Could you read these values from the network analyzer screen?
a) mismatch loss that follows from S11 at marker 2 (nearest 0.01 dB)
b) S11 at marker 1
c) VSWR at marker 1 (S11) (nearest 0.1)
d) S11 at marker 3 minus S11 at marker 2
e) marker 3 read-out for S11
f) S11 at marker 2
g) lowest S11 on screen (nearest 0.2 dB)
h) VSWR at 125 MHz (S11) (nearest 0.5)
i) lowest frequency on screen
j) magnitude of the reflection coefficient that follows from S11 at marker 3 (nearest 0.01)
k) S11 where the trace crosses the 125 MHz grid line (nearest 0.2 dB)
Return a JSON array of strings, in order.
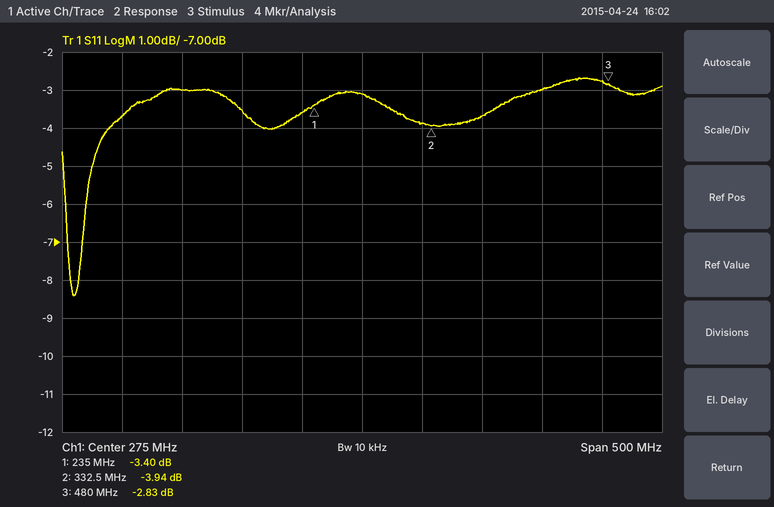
["2.24 dB", "-3.40 dB", "5.2", "1.11 dB", "-2.83 dB", "-3.94 dB", "-8.4 dB", "6.0", "25 MHz", "0.72", "-3.0 dB"]
